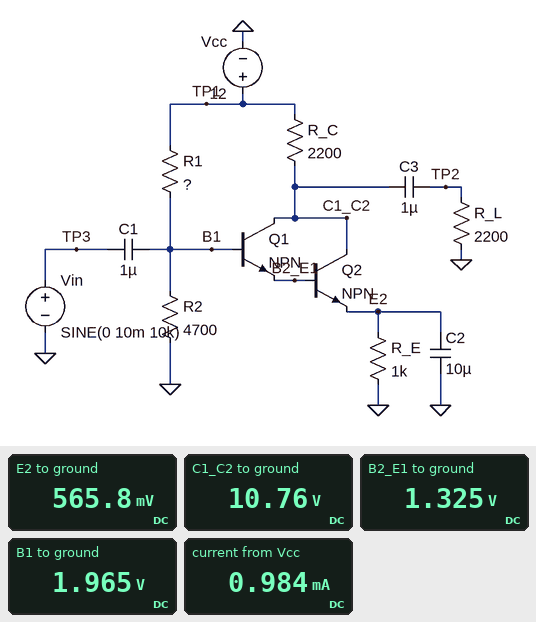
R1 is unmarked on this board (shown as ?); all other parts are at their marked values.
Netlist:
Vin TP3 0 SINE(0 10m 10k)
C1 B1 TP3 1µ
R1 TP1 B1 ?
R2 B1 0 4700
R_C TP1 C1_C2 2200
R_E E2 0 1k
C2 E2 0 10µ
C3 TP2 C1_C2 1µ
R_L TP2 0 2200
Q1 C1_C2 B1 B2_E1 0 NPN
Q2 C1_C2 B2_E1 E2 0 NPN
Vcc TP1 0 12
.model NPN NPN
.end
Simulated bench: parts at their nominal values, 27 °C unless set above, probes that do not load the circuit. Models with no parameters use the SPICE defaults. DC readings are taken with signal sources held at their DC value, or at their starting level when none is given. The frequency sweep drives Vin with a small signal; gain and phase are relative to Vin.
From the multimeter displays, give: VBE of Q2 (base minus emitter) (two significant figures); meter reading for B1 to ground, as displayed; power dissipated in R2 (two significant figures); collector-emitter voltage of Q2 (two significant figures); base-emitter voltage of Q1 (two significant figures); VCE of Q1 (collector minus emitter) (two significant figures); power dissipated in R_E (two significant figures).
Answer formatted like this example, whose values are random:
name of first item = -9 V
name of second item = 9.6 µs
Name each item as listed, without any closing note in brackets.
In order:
VBE of Q2 (base minus emitter) = 760 mV
meter reading for B1 to ground, as displayed = 1.965 V
power dissipated in R2 = 820 µW
collector-emitter voltage of Q2 = 10 V
base-emitter voltage of Q1 = 640 mV
VCE of Q1 (collector minus emitter) = 9.4 V
power dissipated in R_E = 320 µW
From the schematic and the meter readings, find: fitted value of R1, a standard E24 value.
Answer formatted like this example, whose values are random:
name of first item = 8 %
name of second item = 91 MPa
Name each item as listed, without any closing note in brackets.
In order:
fitted value of R1, a standard E24 value = 24 kΩ
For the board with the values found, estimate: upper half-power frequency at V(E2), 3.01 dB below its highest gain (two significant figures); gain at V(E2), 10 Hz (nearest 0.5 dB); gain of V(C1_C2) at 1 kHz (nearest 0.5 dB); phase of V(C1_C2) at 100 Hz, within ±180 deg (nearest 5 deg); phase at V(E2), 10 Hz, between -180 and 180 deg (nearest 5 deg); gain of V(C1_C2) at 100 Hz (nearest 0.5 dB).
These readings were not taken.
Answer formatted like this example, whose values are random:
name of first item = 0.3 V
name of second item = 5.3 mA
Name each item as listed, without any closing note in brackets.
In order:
upper half-power frequency at V(E2), 3.01 dB below its highest gain = 260 Hz
gain at V(E2), 10 Hz = -13.0 dB
gain of V(C1_C2) at 1 kHz = 21.5 dB
phase of V(C1_C2) at 100 Hz, within ±180 deg = -120 deg
phase at V(E2), 10 Hz, between -180 and 180 deg = 75 deg
gain of V(C1_C2) at 100 Hz = 15.5 dB
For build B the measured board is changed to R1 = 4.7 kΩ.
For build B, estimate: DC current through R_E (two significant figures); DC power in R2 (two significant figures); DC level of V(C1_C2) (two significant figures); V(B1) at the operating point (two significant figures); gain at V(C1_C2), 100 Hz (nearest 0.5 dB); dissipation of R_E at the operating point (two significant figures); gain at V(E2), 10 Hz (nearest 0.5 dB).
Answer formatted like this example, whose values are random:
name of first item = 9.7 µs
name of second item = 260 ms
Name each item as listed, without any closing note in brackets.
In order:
DC current through R_E = 3.7 mA
DC power in R2 = 5.9 mW
DC level of V(C1_C2) = 4.5 V
V(B1) at the operating point = 5.3 V
gain at V(C1_C2), 100 Hz = -22.0 dB
dissipation of R_E at the operating point = 14 mW
gain at V(E2), 10 Hz = -30.5 dB
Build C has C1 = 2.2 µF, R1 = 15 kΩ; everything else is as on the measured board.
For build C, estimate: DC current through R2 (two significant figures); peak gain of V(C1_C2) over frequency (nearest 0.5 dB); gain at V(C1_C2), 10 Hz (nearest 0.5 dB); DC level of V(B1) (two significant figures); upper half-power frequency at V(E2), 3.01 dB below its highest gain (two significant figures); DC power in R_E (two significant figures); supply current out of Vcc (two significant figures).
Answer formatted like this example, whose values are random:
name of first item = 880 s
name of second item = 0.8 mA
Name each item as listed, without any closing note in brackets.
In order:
DC current through R2 = 610 µA
peak gain of V(C1_C2) over frequency = 29.5 dB
gain at V(C1_C2), 10 Hz = 0.5 dB
DC level of V(B1) = 2.9 V
upper half-power frequency at V(E2), 3.01 dB below its highest gain = 490 Hz
DC power in R_E = 2.0 mW
supply current out of Vcc = 2.0 mA
